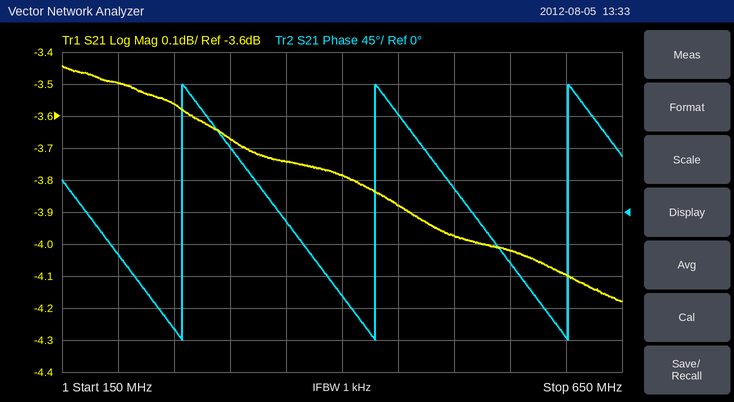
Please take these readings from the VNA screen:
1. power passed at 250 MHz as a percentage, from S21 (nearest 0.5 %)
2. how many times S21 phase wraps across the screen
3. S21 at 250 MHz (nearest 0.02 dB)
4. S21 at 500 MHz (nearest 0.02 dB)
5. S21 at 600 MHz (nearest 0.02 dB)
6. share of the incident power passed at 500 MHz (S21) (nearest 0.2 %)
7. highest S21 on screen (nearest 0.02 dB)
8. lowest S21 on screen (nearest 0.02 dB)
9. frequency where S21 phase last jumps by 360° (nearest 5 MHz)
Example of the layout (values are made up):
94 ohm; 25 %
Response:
44.0 %; 3; -3.56 dB; -3.98 dB; -4.10 dB; 40.0 %; -3.44 dB; -4.18 dB; 600 MHz
